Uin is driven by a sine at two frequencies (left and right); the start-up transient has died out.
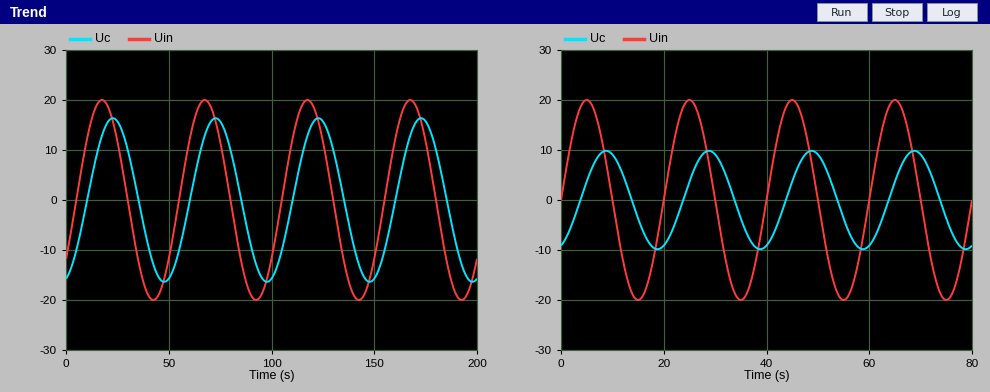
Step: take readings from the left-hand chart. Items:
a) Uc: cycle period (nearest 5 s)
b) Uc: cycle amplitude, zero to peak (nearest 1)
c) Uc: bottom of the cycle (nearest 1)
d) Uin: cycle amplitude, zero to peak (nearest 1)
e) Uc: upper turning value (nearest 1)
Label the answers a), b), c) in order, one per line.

a) 50 s
b) 16
c) -16
d) 20
e) 16
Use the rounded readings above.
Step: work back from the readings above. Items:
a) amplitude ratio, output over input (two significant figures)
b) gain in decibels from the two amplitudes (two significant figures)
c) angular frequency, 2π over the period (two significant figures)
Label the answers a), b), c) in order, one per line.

a) 0.80
b) -1.9 dB
c) 0.13 rad/s
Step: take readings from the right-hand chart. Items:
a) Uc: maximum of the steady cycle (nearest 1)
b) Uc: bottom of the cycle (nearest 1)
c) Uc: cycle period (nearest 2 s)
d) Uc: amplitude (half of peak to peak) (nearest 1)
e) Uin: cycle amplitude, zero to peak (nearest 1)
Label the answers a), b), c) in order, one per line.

a) 10
b) -10
c) 20 s
d) 10
e) 20
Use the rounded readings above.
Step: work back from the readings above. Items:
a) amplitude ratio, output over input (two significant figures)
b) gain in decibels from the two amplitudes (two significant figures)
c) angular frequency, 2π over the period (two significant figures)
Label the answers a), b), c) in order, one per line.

a) 0.50
b) -6.0 dB
c) 0.31 rad/s
